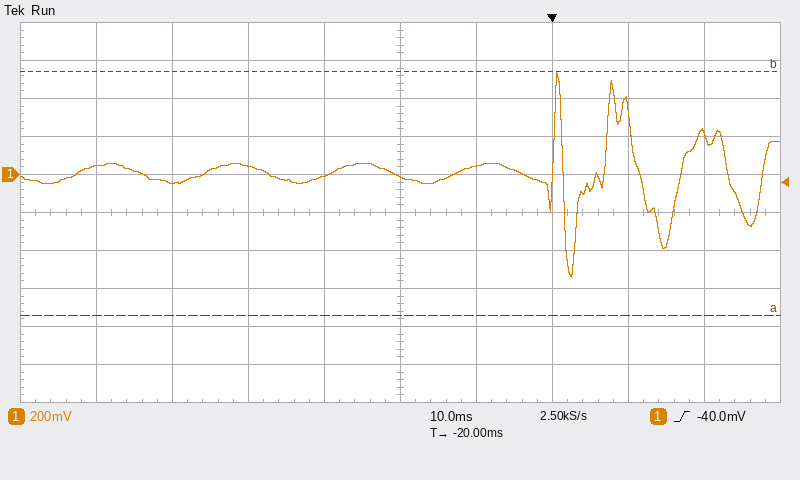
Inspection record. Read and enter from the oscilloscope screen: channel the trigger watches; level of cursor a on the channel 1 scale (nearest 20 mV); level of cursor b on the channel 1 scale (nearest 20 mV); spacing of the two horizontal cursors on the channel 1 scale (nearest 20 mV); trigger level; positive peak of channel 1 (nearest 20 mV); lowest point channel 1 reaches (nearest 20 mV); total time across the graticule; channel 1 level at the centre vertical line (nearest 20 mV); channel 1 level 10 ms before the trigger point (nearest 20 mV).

channel 1
-740 mV
540 mV
1.28 V
-40.0 mV
540 mV
-540 mV
100 ms
-20 mV
40 mV
